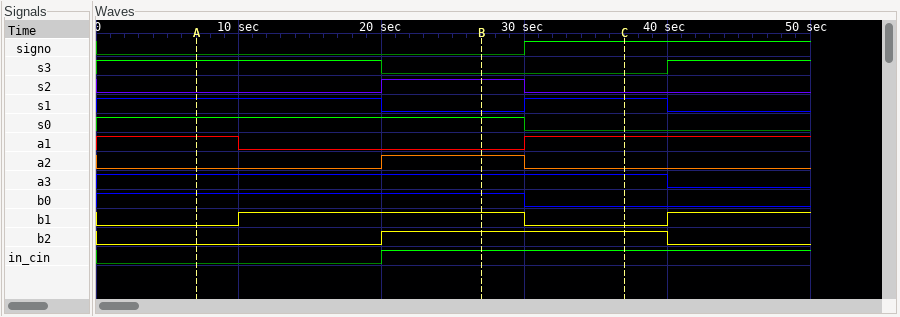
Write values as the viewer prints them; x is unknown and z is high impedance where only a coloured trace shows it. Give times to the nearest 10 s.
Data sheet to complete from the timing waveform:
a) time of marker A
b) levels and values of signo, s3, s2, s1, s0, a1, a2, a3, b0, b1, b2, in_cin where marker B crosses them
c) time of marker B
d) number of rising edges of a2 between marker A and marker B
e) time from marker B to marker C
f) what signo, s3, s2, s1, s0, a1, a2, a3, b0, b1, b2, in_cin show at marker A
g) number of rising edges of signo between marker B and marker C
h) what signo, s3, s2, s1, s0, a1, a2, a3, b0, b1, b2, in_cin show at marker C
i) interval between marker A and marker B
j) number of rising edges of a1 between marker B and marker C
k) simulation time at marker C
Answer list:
10 s
signo=0, s3=0, s2=1, s1=0, s0=1, a1=0, a2=1, a3=1, b0=1, b1=1, b2=1, in_cin=1
30 s
1
10 s
signo=0, s3=1, s2=0, s1=1, s0=1, a1=1, a2=0, a3=1, b0=1, b1=0, b2=0, in_cin=0
1
signo=1, s3=0, s2=0, s1=1, s0=0, a1=1, a2=0, a3=1, b0=0, b1=0, b2=1, in_cin=1
20 s
1
40 s
